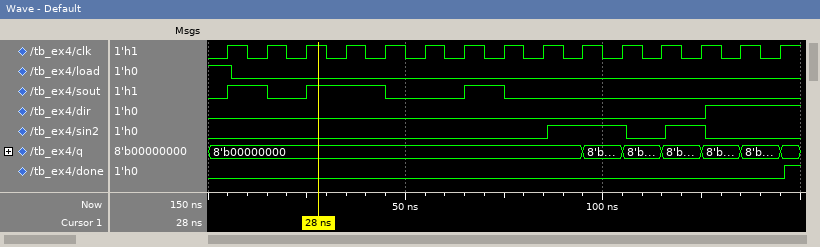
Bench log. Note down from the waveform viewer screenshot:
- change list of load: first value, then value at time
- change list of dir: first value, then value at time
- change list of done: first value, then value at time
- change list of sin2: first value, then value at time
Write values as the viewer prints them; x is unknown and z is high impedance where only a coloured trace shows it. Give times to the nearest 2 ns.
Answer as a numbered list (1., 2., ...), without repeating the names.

1. 1, 0 at 6 ns
2. 0, 1 at 126 ns
3. 0, 1 at 146 ns
4. 0, 1 at 86 ns, 0 at 106 ns, 1 at 116 ns, 0 at 126 ns
